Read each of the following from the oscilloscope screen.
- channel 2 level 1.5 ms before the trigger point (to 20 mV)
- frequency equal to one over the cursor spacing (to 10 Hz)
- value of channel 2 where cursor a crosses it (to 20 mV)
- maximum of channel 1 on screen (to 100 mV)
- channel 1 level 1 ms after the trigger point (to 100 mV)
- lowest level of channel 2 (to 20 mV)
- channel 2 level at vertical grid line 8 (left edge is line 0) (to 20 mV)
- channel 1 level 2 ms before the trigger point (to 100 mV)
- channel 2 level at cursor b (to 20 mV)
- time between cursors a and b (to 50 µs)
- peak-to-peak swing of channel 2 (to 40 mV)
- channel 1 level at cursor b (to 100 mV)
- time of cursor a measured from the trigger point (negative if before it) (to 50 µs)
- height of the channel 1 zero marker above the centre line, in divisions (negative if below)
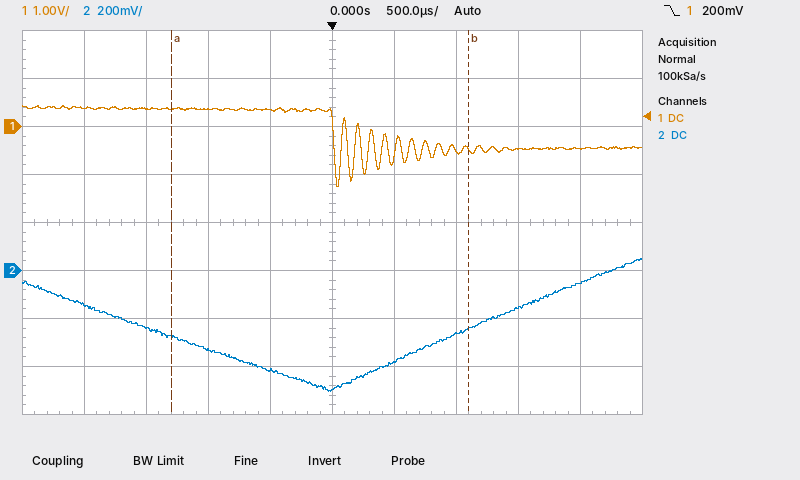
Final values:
-240 mV
420 Hz
-280 mV
400 mV
-500 mV
-500 mV
-160 mV
400 mV
-240 mV
2.40 ms
560 mV
-500 mV
-1.30 ms
+2.0 div
